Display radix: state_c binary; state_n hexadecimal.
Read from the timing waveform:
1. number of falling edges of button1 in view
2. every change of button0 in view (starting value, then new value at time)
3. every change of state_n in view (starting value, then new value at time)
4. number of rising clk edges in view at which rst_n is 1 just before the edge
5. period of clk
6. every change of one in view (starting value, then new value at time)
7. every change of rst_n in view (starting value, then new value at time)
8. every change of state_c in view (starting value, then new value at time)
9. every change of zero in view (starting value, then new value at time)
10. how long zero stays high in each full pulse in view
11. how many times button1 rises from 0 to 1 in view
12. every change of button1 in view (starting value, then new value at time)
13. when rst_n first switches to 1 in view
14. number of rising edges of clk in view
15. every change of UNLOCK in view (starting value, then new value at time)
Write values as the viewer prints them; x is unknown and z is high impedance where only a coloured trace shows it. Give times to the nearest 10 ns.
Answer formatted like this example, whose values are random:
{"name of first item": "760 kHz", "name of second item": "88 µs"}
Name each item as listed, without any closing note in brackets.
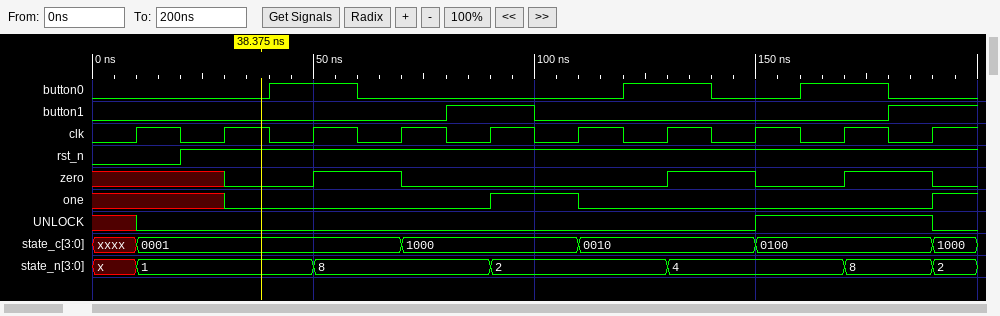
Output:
{"number of falling edges of button1 in view": "1", "every change of button0 in view": "0, 1 at 40 ns, 0 at 60 ns, 1 at 120 ns, 0 at 140 ns, 1 at 160 ns, 0 at 180 ns", "every change of state_n in view": "x, 1 at 10 ns, 8 at 50 ns, 2 at 90 ns, 4 at 130 ns, 8 at 170 ns, 2 at 190 ns", "number of rising clk edges in view at which rst_n is 1 just before the edge": "9", "period of clk": "20 ns", "every change of one in view": "x, 0 at 30 ns, 1 at 90 ns, 0 at 110 ns, 1 at 190 ns", "every change of rst_n in view": "0, 1 at 20 ns", "every change of state_c in view": "xxxx, 0001 at 10 ns, 1000 at 70 ns, 0010 at 110 ns, 0100 at 150 ns, 1000 at 190 ns", "every change of zero in view": "x, 0 at 30 ns, 1 at 50 ns, 0 at 70 ns, 1 at 130 ns, 0 at 150 ns, 1 at 170 ns, 0 at 190 ns", "how long zero stays high in each full pulse in view": "20 ns, 20 ns, 20 ns", "how many times button1 rises from 0 to 1 in view": "2", "every change of button1 in view": "0, 1 at 80 ns, 0 at 100 ns, 1 at 180 ns", "when rst_n first switches to 1 in view": "20 ns", "number of rising edges of clk in view": "10", "every change of UNLOCK in view": "x, 0 at 10 ns, 1 at 150 ns, 0 at 190 ns"}
